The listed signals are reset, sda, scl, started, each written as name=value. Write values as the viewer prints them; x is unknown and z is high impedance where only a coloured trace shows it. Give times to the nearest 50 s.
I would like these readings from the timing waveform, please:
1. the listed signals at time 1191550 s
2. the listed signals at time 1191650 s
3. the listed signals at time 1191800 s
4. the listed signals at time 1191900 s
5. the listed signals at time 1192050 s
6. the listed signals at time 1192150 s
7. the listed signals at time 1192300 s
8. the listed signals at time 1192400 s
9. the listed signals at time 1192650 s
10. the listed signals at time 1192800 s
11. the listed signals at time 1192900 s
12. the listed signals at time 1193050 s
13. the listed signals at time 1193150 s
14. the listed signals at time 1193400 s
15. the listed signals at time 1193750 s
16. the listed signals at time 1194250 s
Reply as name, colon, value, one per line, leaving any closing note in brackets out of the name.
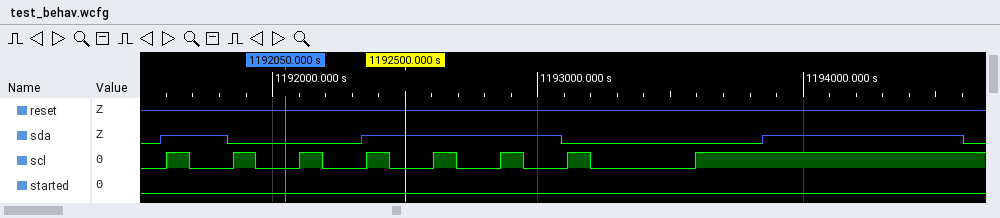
the listed signals at time 1191550 s: reset=z, sda=0, scl=0, started=0
the listed signals at time 1191650 s: reset=z, sda=z, scl=1, started=0
the listed signals at time 1191800 s: reset=z, sda=z, scl=0, started=0
the listed signals at time 1191900 s: reset=z, sda=0, scl=1, started=0
the listed signals at time 1192050 s: reset=z, sda=0, scl=0, started=0
the listed signals at time 1192150 s: reset=z, sda=0, scl=1, started=0
the listed signals at time 1192300 s: reset=z, sda=0, scl=0, started=0
the listed signals at time 1192400 s: reset=z, sda=z, scl=1, started=0
the listed signals at time 1192650 s: reset=z, sda=z, scl=1, started=0
the listed signals at time 1192800 s: reset=z, sda=z, scl=0, started=0
the listed signals at time 1192900 s: reset=z, sda=z, scl=1, started=0
the listed signals at time 1193050 s: reset=z, sda=z, scl=0, started=0
the listed signals at time 1193150 s: reset=z, sda=0, scl=1, started=0
the listed signals at time 1193400 s: reset=z, sda=0, scl=0, started=0
the listed signals at time 1193750 s: reset=z, sda=0, scl=1, started=0
the listed signals at time 1194250 s: reset=z, sda=z, scl=1, started=0
